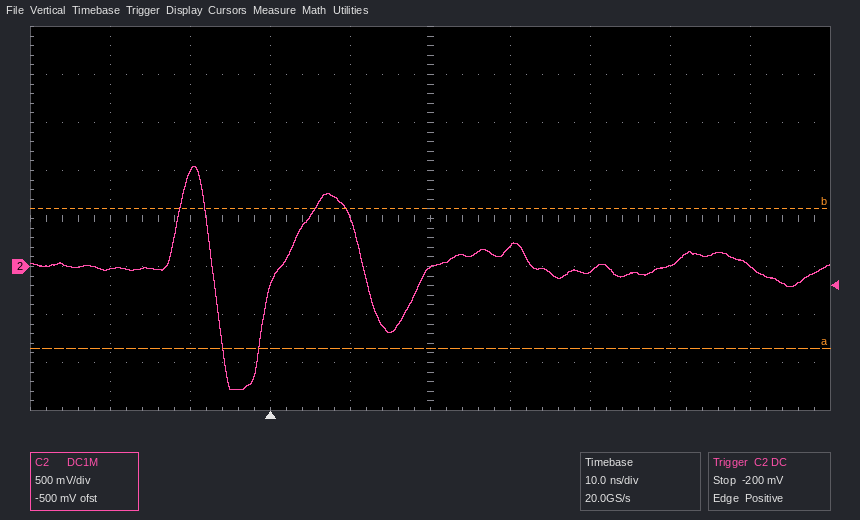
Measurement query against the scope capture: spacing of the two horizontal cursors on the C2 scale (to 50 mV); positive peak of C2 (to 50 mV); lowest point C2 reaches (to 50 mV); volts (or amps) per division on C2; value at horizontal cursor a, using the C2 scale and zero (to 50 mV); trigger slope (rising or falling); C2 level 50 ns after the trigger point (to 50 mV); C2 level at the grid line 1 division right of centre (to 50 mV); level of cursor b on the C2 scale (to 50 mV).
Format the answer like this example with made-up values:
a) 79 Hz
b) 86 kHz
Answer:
a) 1.45 V
b) 1.05 V
c) -1.30 V
d) 500 mV
e) -850 mV
f) rising
g) 0 mV
h) 200 mV
i) 600 mV
